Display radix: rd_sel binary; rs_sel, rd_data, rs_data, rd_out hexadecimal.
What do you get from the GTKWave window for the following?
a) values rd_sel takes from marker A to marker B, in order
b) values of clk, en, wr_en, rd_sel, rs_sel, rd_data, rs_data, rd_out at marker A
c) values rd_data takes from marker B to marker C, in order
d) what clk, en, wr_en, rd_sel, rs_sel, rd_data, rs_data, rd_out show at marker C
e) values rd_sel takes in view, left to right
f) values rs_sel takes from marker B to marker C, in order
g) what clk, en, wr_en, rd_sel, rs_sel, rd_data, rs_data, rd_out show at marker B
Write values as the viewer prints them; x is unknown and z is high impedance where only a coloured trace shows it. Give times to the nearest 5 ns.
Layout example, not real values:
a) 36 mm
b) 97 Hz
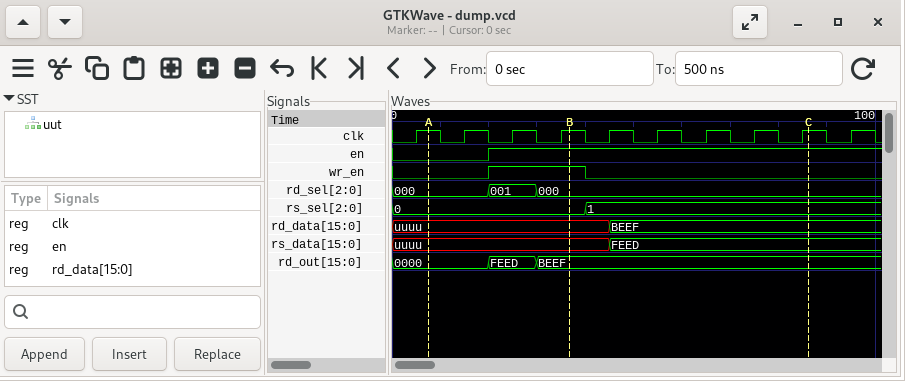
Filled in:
a) 000, 001, 000
b) clk=1, en=0, wr_en=0, rd_sel=000, rs_sel=0, rd_data=uuuu, rs_data=uuuu, rd_out=0000
c) uuuu, BEEF
d) clk=1, en=1, wr_en=0, rd_sel=000, rs_sel=1, rd_data=BEEF, rs_data=FEED, rd_out=BEEF
e) 000, 001, 000
f) 0, 1
g) clk=1, en=1, wr_en=1, rd_sel=000, rs_sel=0, rd_data=uuuu, rs_data=uuuu, rd_out=BEEF
